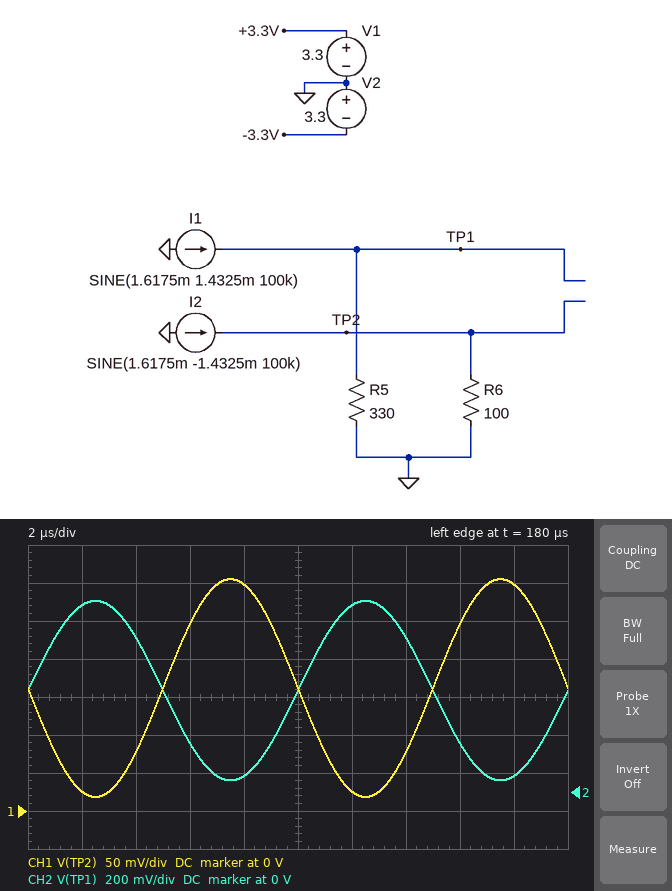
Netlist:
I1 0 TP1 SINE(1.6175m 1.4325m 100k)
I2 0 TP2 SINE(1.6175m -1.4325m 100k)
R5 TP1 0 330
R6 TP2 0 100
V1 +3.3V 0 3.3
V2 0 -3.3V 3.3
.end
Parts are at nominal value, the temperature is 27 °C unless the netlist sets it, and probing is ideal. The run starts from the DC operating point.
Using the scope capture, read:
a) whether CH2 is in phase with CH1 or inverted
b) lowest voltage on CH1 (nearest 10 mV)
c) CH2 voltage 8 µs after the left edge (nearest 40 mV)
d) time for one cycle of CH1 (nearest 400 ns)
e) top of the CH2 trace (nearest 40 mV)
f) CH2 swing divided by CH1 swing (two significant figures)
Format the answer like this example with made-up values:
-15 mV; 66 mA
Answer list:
inverted; 20 mV; 80 mV; 10.0 µs; 1.00 V; 3.3
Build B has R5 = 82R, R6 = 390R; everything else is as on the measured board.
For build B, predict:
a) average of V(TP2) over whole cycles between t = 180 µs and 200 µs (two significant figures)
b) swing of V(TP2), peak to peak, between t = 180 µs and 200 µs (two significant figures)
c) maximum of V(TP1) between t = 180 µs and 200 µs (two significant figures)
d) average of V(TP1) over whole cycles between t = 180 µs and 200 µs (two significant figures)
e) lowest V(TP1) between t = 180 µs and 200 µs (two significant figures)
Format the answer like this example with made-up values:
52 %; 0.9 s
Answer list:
630 mV; 1.1 V; 250 mV; 130 mV; 15 mV
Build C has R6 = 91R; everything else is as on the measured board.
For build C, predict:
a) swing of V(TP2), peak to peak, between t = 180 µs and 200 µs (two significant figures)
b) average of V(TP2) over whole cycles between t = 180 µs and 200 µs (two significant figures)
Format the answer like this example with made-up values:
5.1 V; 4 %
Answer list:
260 mV; 150 mV
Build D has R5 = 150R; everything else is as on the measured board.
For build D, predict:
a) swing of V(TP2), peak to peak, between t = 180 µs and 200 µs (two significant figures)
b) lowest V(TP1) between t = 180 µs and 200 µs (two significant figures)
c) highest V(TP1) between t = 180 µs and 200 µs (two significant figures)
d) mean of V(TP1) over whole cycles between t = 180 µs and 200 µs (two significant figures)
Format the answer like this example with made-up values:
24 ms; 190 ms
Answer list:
290 mV; 28 mV; 460 mV; 240 mV
